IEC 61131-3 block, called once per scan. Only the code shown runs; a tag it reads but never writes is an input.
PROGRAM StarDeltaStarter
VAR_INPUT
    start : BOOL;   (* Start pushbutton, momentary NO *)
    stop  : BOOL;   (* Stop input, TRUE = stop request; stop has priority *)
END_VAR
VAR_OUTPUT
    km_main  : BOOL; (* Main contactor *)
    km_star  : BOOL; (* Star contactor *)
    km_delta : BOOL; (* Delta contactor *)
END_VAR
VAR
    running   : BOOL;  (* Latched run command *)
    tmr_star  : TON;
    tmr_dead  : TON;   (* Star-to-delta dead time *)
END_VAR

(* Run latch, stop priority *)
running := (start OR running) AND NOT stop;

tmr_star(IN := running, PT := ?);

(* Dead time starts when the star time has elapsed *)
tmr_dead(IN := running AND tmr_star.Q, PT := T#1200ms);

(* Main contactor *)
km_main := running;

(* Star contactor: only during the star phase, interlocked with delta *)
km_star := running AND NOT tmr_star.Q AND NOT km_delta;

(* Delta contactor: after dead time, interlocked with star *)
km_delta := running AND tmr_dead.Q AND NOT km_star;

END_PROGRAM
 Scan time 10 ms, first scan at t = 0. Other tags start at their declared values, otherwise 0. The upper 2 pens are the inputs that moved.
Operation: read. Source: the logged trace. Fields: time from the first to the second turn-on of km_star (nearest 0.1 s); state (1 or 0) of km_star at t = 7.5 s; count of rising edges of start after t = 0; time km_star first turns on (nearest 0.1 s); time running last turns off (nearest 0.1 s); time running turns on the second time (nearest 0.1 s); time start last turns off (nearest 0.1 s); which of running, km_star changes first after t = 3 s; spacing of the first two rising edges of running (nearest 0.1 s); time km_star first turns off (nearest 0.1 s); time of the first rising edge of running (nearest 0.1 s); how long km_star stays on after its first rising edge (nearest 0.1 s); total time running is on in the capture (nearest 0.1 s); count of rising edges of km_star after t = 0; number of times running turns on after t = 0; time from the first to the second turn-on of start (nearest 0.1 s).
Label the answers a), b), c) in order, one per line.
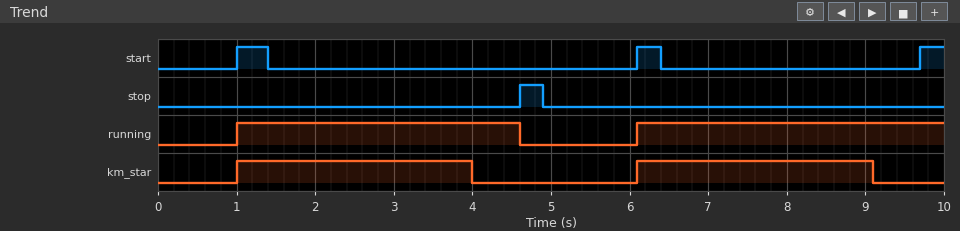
a) 5.1 s
b) 1
c) 3
d) 1.0 s
e) 4.6 s
f) 6.1 s
g) 6.4 s
h) km_star
i) 5.1 s
j) 4.0 s
k) 1.0 s
l) 3.0 s
m) 7.5 s
n) 2
o) 2
p) 5.1 s
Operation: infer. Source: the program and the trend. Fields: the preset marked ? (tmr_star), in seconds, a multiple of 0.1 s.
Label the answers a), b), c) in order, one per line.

a) 3.0 s
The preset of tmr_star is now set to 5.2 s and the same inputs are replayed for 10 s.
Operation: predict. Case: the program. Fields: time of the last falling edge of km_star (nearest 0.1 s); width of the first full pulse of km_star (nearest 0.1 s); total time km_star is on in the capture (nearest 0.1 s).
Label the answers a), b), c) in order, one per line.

a) 4.6 s
b) 3.6 s
c) 7.5 s
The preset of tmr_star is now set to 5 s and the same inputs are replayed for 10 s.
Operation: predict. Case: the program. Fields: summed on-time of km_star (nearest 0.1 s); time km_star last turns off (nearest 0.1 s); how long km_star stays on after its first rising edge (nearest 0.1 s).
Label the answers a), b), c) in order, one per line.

a) 7.5 s
b) 4.6 s
c) 3.6 s
